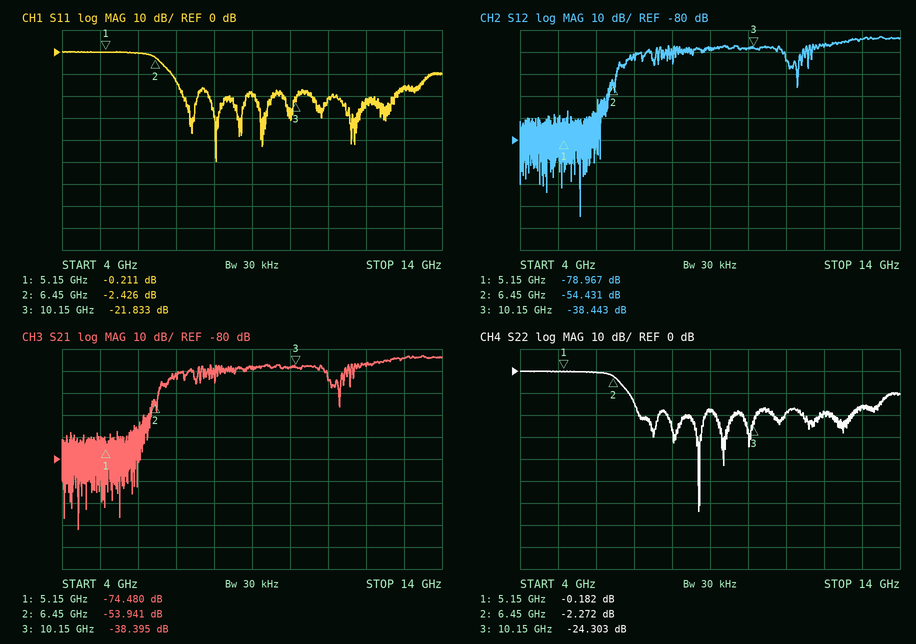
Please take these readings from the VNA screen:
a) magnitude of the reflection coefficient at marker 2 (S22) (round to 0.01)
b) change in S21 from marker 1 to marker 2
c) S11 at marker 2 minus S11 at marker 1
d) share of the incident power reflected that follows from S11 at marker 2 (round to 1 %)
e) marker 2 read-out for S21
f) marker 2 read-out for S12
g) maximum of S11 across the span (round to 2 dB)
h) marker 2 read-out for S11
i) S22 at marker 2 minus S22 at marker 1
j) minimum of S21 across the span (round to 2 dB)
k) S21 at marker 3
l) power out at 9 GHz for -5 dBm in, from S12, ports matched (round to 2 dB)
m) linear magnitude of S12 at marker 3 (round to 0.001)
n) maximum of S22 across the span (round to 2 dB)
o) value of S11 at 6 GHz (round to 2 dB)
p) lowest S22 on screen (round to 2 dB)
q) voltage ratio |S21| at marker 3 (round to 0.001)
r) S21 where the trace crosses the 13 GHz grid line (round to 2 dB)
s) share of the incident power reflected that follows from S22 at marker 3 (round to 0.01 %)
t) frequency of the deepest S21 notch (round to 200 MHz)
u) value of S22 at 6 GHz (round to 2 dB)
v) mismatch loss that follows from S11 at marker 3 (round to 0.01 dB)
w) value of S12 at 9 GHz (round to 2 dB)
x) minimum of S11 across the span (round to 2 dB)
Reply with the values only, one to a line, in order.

0.77
20.539 dB
-2.215 dB
57 %
-53.941 dB
-54.431 dB
0 dB
-2.426 dB
-2.090 dB
-112 dB
-38.395 dB
-44 dBm
0.012
0 dB
0 dB
-64 dB
0.012
-34 dB
0.37 %
4.4 GHz
0 dB
0.03 dB
-38 dB
-50 dB
